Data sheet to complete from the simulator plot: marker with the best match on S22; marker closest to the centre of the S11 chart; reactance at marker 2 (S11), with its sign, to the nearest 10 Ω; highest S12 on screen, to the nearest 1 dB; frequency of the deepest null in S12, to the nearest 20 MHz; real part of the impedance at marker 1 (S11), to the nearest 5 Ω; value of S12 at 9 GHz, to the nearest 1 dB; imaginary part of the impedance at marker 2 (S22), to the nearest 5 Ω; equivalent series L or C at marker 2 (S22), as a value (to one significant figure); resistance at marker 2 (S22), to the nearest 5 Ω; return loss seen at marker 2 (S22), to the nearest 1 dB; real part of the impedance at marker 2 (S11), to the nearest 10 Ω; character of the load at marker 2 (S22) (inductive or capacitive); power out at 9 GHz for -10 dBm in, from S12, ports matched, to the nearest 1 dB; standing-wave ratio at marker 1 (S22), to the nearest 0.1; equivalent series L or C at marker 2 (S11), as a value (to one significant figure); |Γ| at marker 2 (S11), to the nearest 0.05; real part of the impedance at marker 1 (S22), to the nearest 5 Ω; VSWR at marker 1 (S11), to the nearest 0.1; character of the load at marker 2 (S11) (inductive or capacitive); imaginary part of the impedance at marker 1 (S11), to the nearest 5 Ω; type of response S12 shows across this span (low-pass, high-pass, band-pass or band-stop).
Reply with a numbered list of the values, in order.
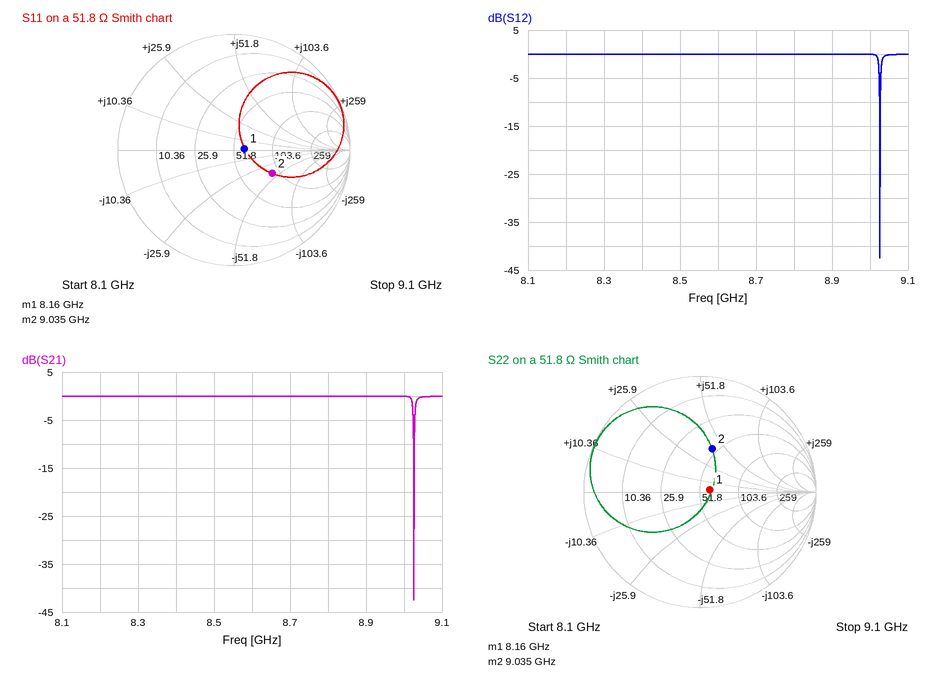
1. marker 1
2. marker 1
3. -40 Ω
4. 0 dB
5. 9.02 GHz
6. 60 Ω
7. 0 dB
8. +40 Ω
9. 700 pH
10. 45 Ω
11. 8 dB
12. 90 Ω
13. inductive
14. -10 dBm
15. 1.2
16. 400 fF
17. 0.40
18. 60 Ω
19. 1.2
20. capacitive
21. 0 Ω
22. band-stop
